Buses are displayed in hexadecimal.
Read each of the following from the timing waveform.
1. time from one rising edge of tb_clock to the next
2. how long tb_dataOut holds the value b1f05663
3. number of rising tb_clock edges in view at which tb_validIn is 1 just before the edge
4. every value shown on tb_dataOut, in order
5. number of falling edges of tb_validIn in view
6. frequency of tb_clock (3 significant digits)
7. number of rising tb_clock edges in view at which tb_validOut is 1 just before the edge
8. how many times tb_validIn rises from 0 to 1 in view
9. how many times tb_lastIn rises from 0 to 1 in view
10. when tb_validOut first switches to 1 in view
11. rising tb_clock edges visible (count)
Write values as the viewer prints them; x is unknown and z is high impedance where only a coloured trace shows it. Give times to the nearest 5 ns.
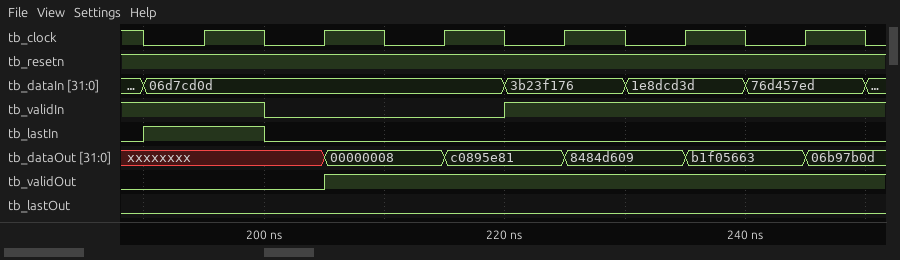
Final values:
10 ns
10 ns
4
xxxxxxxx, 00000008, c0895e81, 8484d609, b1f05663, 06b97b0d
1
100 MHz
4
1
1
205 ns
6
